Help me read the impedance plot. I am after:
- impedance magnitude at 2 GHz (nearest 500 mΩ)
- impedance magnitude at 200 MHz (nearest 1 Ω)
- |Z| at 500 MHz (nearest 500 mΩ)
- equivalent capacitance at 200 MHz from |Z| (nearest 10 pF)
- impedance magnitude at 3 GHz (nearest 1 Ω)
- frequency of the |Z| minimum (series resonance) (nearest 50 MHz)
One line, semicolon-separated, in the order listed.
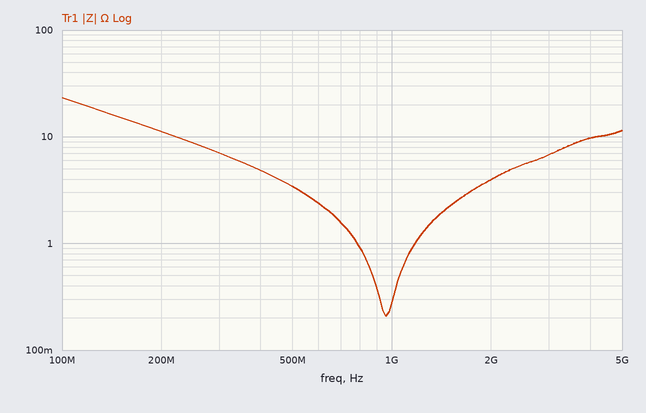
4.0 Ω; 11 Ω; 3.5 Ω; 70 pF; 7 Ω; 950 MHz
